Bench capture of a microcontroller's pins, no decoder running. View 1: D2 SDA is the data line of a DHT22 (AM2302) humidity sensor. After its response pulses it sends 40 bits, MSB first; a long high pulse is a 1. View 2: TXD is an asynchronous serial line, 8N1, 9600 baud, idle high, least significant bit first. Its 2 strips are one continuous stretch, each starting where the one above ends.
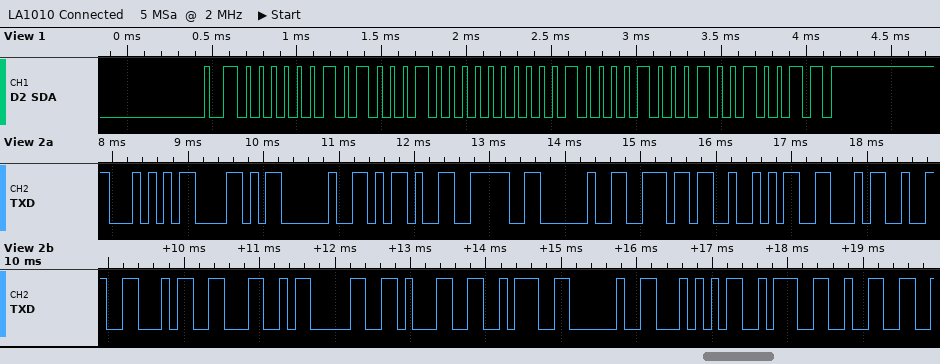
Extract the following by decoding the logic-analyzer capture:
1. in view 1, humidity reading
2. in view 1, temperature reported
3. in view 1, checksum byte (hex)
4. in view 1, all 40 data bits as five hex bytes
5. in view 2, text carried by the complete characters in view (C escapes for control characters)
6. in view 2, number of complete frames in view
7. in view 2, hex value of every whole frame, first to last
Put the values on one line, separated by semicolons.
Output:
64.8 %; 26.4 °C; 0x93; 02 88 01 08 93; "TX -> nRF24L01: T:2"; 19; 54 58 20 2D 3E 20 6E 52 46 32 34 4C 30 31 3A 20 54 3A 32
